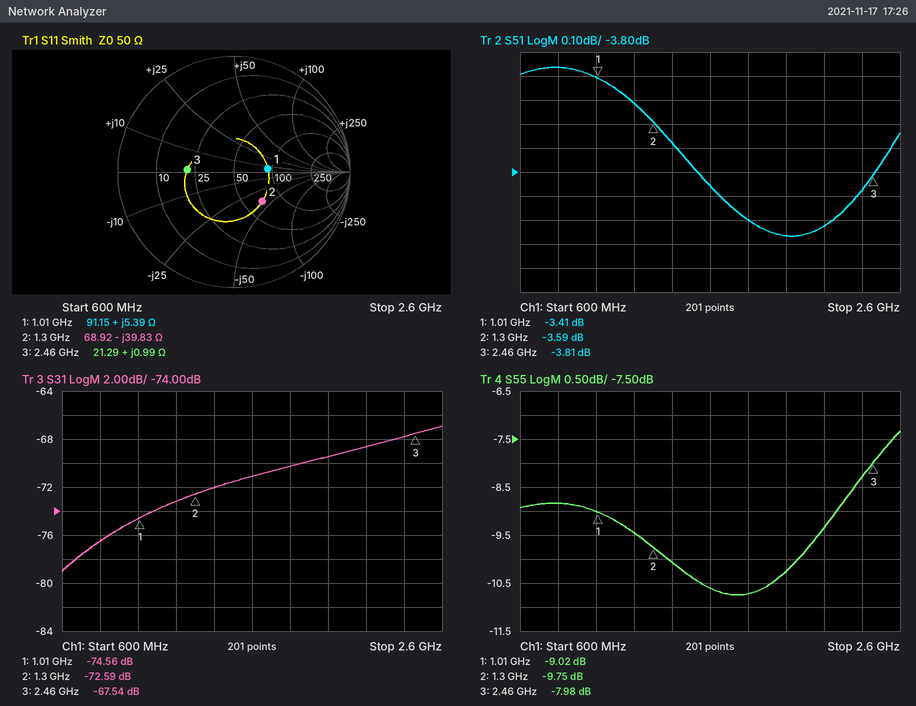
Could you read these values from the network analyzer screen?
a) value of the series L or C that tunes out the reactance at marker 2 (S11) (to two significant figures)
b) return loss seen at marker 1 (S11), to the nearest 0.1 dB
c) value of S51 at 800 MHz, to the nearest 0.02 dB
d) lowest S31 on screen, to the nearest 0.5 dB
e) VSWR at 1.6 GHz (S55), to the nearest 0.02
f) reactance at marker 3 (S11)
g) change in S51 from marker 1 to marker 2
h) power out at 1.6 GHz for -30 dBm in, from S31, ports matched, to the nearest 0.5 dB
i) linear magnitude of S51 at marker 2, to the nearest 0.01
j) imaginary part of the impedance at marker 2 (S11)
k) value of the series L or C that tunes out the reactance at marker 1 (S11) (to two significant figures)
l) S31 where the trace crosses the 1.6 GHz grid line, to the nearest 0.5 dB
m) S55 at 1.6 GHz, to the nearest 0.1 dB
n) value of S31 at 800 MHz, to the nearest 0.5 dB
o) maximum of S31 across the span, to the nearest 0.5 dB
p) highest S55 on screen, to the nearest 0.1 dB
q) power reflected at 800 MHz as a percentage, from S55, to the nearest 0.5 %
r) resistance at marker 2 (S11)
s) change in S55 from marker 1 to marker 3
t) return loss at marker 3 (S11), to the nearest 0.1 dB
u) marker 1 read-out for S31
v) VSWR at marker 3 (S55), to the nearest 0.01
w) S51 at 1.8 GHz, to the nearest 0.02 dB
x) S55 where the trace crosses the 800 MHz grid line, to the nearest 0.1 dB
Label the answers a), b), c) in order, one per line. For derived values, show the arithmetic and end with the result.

a) L = 39.83 Ω/(2π × 1.3 GHz) ≈ 4.9 nH
b) 10.6 dB
c) -3.36 dB
d) -79.0 dB
e) |Γ| = 10^(-10.6/20) = 0.2951; VSWR = (1 + 0.2951)/(1 − 0.2951) ≈ 1.84
f) +0.99 Ω
g) -3.59 − (-3.41) = -0.18 dB
h) -30 dBm + (-71.0 dB) = -101.0 dBm
i) 10^(-3.59/20) ≈ 0.66
j) -39.83 Ω
k) C = 1/(2π × 1.01 GHz × 5.39 Ω) ≈ 29 pF
l) -71.0 dB
m) -10.6 dB
n) -76.5 dB
o) -67.0 dB
p) -7.3 dB
q) 10^(-8.8/10) ≈ 13.2 %, so 13.0 % to the nearest 0.5 %
r) 68.92 Ω
s) -7.98 − (-9.02) = 1.04 dB
t) 7.9 dB
u) -74.56 dB
v) (1 + 0.3990)/(1 − 0.3990) ≈ 2.33
w) -4.00 dB
x) -8.8 dB
